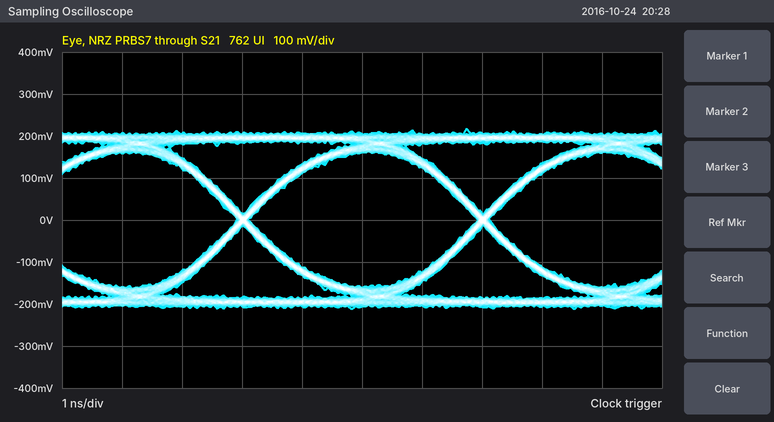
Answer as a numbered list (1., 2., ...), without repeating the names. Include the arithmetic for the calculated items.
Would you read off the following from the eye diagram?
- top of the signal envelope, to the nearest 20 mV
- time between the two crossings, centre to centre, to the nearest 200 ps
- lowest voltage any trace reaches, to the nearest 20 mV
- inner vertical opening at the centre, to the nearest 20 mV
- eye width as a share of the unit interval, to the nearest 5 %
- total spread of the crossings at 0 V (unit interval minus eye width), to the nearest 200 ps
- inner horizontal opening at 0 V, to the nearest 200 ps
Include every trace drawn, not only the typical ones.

1. 220 mV
2. 4.0 ns
3. -220 mV
4. 320 mV
5. 3.8 ns / 4.0 ns ≈ 95 %
6. 200 ps
7. 3.8 ns
